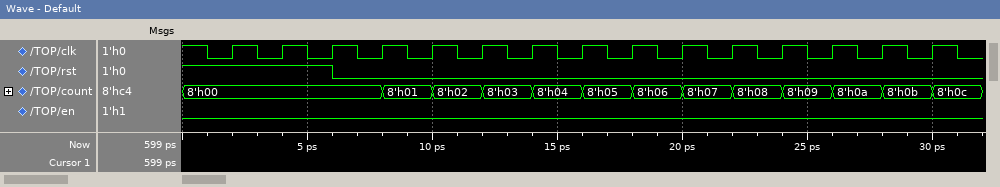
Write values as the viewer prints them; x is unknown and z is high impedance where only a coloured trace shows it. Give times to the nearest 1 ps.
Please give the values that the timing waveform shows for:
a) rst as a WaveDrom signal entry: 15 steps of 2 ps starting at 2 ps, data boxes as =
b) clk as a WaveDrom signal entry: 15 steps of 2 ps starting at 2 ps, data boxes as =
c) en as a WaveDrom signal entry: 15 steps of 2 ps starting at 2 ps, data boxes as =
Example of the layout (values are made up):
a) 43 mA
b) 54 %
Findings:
a) {name: 'rst', wave: '1.0............'}
b) {name: 'clk', wave: 'p..............'}
c) {name: 'en', wave: '0..............'}
